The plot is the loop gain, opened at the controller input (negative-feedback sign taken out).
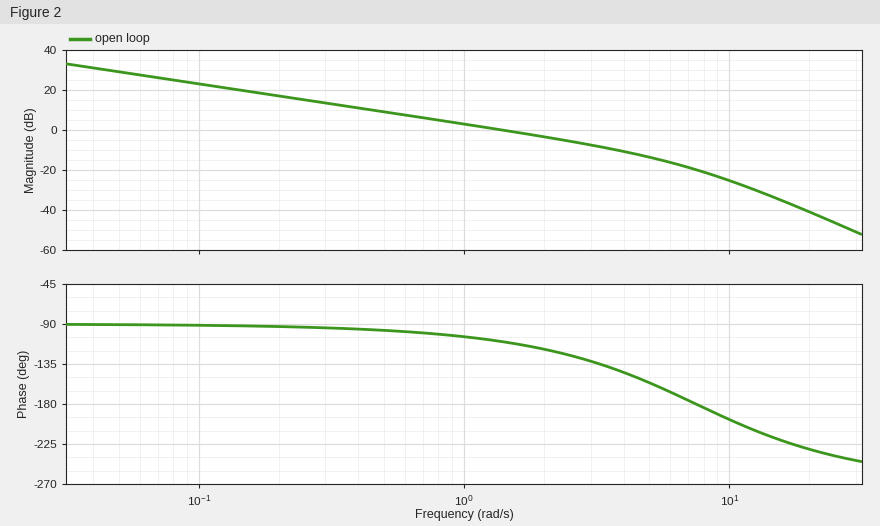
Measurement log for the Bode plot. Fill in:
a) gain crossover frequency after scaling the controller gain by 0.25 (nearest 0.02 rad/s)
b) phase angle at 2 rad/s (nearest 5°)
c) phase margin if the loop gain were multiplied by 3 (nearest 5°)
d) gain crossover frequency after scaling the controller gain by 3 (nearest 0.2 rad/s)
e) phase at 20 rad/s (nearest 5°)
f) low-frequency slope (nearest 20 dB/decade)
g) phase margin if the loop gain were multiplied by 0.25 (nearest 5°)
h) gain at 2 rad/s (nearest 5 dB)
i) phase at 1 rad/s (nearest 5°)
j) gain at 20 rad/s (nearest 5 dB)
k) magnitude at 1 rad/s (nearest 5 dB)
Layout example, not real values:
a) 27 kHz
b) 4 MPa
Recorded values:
a) 0.36 rad/s
b) -120°
c) 40°
d) 3.6 rad/s
e) -230°
f) -20 dB/decade
g) 85°
h) -5 dB
i) -105°
j) -40 dB
k) 5 dB
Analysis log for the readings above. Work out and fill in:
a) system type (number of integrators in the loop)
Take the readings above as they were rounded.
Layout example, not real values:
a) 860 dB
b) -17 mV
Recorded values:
a) 1
